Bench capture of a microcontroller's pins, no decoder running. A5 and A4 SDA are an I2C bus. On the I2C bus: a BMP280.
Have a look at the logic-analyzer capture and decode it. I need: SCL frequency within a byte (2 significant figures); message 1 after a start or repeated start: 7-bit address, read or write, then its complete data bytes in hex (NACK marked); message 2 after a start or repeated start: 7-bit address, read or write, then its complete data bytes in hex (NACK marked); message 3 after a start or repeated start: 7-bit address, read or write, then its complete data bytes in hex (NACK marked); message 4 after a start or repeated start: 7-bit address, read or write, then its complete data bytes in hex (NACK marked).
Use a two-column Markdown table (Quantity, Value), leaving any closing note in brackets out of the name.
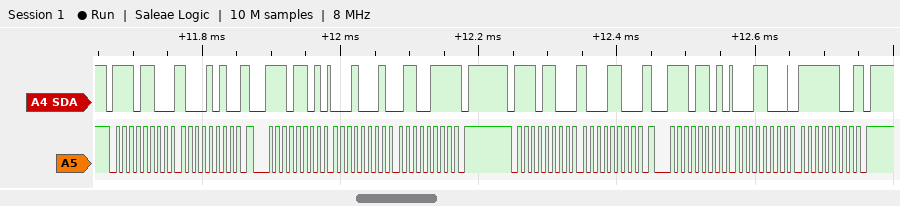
| Quantity | Value |
|---|---|
| SCL frequency within a byte | 100 kHz |
| message 1 after a start or repeated start: 7-bit address, read or write, then its complete data bytes in hex | 0x76 write: 8A |
| message 2 after a start or repeated start: 7-bit address, read or write, then its complete data bytes in hex | 0x76 read: 11 67 NACK |
| message 3 after a start or repeated start: 7-bit address, read or write, then its complete data bytes in hex | 0x76 write: 8C |
| message 4 after a start or repeated start: 7-bit address, read or write, then its complete data bytes in hex | 0x76 read: 18 FC NACK |
